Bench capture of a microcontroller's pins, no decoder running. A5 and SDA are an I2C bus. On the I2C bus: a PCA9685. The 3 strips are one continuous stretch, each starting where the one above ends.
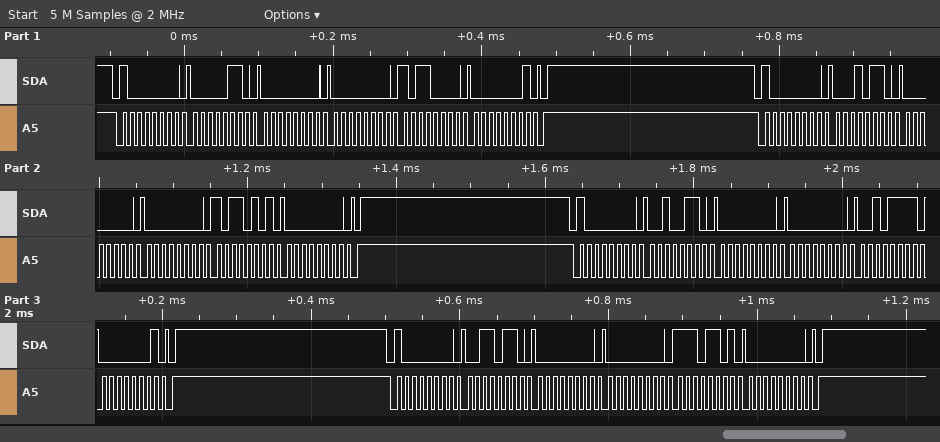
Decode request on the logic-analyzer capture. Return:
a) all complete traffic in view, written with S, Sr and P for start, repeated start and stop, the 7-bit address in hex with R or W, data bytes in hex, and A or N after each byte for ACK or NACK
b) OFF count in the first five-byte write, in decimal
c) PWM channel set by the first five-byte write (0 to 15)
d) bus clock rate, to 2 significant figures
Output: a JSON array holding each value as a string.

["S 40W A 06 A 00 A 00 A B0 A 01 A P S 40W A 16 A 00 A 00 A B5 A 00 A P S 40W A 26 A 00 A 00 A 2F A 01 A P S 40W A 36 A 00 A 00 A ED A 00 A P", "432", "0", "100 kHz"]
